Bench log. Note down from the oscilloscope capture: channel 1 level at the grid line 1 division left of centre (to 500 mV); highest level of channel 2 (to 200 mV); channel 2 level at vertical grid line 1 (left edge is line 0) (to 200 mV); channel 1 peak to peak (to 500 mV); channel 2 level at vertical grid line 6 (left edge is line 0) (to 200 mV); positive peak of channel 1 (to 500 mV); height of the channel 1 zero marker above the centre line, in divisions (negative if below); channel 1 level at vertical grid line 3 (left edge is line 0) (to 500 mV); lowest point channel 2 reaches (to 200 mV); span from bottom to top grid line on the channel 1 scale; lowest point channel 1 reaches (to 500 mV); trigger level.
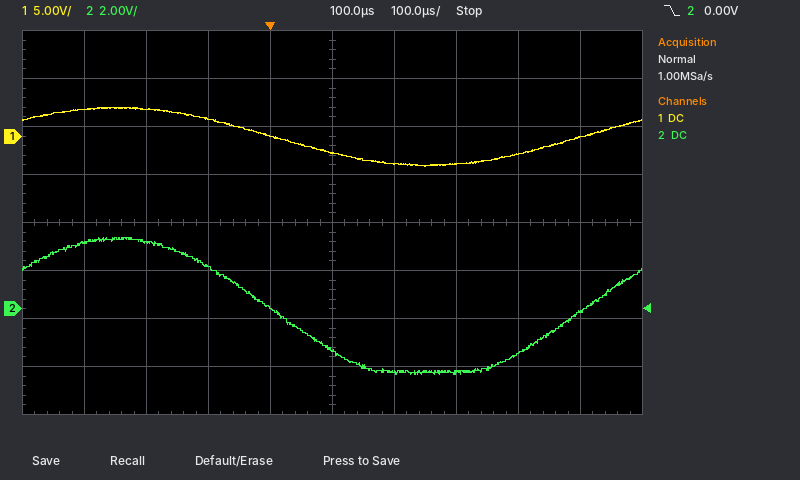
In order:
0.0 V
3.0 V
2.8 V
6.0 V
-2.6 V
3.0 V
+1.8 div
2.0 V
-2.8 V
40 V
-3.0 V
0.00 V
